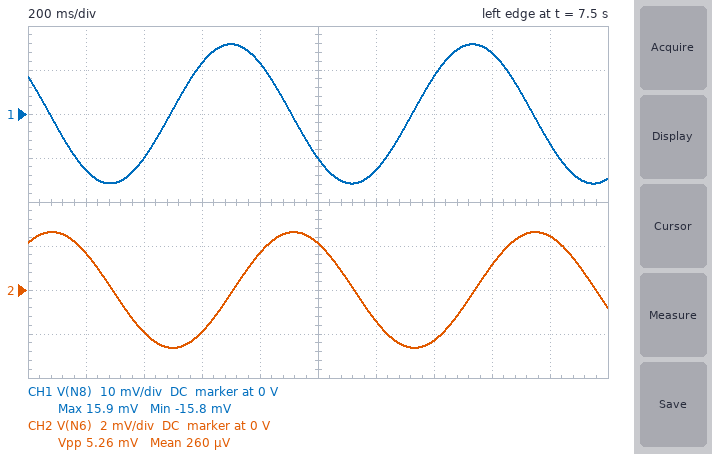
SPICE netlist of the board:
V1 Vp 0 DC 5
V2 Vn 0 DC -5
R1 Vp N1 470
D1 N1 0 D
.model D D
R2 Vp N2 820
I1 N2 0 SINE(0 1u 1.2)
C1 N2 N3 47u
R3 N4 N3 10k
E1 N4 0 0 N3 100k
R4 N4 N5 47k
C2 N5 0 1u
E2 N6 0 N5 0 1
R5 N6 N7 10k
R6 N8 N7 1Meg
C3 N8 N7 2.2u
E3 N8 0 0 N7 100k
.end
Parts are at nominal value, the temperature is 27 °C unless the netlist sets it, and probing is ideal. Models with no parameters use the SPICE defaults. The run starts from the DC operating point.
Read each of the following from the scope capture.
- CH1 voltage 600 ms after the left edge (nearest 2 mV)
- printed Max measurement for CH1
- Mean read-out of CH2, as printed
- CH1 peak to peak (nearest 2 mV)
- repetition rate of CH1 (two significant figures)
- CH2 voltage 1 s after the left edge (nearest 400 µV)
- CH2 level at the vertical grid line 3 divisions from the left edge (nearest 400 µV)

12 mV
15.9 mV
260 µV
32 mV
1.2 Hz
2.0 mV
-2.0 mV
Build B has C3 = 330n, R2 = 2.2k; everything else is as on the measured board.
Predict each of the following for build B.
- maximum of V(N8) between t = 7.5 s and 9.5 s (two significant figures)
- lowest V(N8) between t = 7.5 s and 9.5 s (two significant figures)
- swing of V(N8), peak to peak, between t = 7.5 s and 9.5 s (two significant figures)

220 mV
-220 mV
430 mV
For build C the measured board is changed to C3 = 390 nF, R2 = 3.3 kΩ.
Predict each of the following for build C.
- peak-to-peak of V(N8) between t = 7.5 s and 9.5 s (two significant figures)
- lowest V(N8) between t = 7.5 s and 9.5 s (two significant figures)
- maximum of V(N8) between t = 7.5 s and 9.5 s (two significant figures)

460 mV
-230 mV
230 mV
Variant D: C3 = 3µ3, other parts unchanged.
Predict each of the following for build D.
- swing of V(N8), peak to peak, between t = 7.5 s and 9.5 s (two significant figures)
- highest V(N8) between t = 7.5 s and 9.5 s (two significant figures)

21 mV
11 mV
